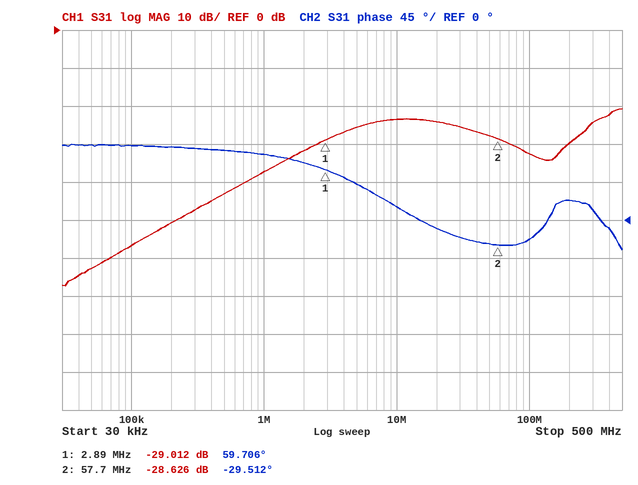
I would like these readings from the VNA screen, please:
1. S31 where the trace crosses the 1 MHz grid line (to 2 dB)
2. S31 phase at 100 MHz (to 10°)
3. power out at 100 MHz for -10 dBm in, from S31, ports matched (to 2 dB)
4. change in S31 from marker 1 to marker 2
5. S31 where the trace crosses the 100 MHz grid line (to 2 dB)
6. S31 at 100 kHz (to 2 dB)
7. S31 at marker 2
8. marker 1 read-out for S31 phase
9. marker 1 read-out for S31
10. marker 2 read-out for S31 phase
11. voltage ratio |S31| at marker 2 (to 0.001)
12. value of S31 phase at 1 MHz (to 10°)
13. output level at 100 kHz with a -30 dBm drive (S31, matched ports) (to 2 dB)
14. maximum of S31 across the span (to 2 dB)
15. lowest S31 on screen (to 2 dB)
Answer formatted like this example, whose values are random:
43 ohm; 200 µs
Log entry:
-38 dB; -20°; -42 dBm; 0.386 dB; -32 dB; -56 dB; -28.626 dB; 59.706°; -29.012 dB; -29.512°; 0.037; 80°; -86 dBm; -20 dB; -68 dB
